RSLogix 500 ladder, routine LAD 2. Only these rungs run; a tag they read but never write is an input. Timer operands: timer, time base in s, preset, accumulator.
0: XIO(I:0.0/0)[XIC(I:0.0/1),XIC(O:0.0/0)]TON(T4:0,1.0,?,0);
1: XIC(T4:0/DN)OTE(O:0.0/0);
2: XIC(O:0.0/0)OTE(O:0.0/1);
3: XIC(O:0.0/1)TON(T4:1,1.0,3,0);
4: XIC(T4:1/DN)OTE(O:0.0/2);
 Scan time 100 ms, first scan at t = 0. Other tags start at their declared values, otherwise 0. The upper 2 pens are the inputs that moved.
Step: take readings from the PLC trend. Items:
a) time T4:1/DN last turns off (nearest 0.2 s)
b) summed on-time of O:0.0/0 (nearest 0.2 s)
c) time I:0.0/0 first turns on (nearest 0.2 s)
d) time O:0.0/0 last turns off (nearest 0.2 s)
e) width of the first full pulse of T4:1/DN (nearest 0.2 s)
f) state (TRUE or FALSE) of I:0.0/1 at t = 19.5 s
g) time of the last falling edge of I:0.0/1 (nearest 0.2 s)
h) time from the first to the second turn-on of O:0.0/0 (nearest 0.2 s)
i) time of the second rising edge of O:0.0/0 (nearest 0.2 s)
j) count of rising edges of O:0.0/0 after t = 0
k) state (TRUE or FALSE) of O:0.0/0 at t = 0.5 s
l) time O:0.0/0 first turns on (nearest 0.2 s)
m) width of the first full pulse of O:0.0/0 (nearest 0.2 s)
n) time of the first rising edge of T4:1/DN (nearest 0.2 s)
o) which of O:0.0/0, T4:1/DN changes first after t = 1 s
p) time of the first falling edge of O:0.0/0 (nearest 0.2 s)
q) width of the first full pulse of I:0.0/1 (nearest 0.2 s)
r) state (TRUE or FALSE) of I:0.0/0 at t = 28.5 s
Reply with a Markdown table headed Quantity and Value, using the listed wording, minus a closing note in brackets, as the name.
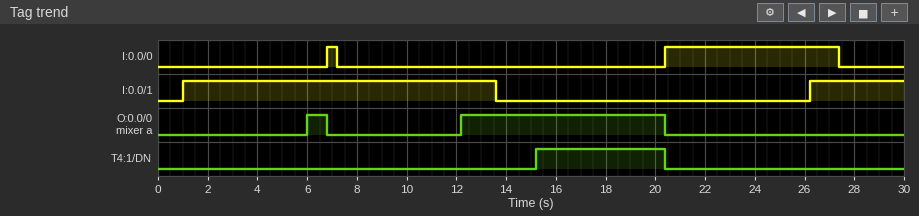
| Quantity | Value |
|---|---|
| time T4:1/DN last turns off | 20.4 s |
| summed on-time of O:0.0/0 | 9.0 s |
| time I:0.0/0 first turns on | 6.8 s |
| time O:0.0/0 last turns off | 20.4 s |
| width of the first full pulse of T4:1/DN | 5.2 s |
| state (TRUE or FALSE) of I:0.0/1 at t = 19.5 s | FALSE |
| time of the last falling edge of I:0.0/1 | 13.6 s |
| time from the first to the second turn-on of O:0.0/0 | 6.2 s |
| time of the second rising edge of O:0.0/0 | 12.2 s |
| count of rising edges of O:0.0/0 after t = 0 | 2 |
| state (TRUE or FALSE) of O:0.0/0 at t = 0.5 s | FALSE |
| time O:0.0/0 first turns on | 6.0 s |
| width of the first full pulse of O:0.0/0 | 0.8 s |
| time of the first rising edge of T4:1/DN | 15.2 s |
| which of O:0.0/0, T4:1/DN changes first after t = 1 s | O:0.0/0 |
| time of the first falling edge of O:0.0/0 | 6.8 s |
| width of the first full pulse of I:0.0/1 | 12.6 s |
| state (TRUE or FALSE) of I:0.0/0 at t = 28.5 s | FALSE |
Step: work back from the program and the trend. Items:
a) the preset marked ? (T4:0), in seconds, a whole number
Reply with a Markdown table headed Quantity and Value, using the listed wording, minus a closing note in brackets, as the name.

| Quantity | Value |
|---|---|
| the preset marked ? (T4:0), in seconds, a whole number | 5 s |
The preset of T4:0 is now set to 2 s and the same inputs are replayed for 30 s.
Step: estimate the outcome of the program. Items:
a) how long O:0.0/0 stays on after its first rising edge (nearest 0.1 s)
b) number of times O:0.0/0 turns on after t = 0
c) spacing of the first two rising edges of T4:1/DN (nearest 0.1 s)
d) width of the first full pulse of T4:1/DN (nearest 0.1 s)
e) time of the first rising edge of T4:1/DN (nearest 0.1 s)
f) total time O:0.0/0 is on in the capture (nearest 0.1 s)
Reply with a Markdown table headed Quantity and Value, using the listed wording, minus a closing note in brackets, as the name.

| Quantity | Value |
|---|---|
| how long O:0.0/0 stays on after its first rising edge | 3.8 s |
| number of times O:0.0/0 turns on after t = 0 | 3 |
| spacing of the first two rising edges of T4:1/DN | 6.2 s |
| width of the first full pulse of T4:1/DN | 0.8 s |
| time of the first rising edge of T4:1/DN | 6.0 s |
| total time O:0.0/0 is on in the capture | 15.6 s |
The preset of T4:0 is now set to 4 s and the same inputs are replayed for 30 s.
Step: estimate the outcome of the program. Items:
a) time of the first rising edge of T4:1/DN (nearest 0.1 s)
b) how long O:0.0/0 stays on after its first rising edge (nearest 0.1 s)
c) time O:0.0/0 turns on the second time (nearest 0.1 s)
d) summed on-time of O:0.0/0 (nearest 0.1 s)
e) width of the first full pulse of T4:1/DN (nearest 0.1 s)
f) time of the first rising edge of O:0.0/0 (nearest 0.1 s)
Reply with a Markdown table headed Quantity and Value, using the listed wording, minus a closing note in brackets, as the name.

| Quantity | Value |
|---|---|
| time of the first rising edge of T4:1/DN | 14.2 s |
| how long O:0.0/0 stays on after its first rising edge | 1.8 s |
| time O:0.0/0 turns on the second time | 11.2 s |
| summed on-time of O:0.0/0 | 11.0 s |
| width of the first full pulse of T4:1/DN | 6.2 s |
| time of the first rising edge of O:0.0/0 | 5.0 s |
